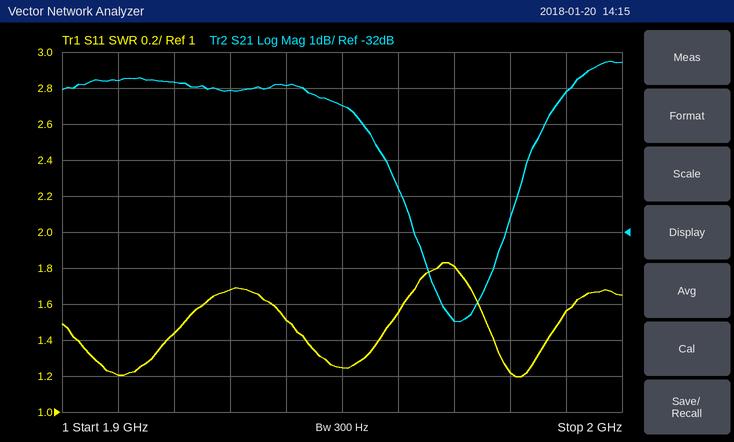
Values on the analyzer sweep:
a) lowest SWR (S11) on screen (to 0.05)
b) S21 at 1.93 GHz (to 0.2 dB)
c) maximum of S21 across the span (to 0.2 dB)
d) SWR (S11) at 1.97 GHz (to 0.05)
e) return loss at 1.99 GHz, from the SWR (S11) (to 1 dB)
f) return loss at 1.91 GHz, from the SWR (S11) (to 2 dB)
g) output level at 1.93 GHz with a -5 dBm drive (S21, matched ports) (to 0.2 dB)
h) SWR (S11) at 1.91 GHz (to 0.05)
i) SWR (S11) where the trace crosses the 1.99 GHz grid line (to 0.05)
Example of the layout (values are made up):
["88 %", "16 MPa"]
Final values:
["1.20", "-28.0 dB", "-27.2 dB", "1.80", "13 dB", "20 dB", "-33.0 dBm", "1.20", "1.55"]
